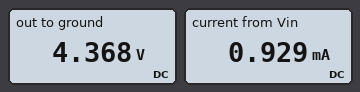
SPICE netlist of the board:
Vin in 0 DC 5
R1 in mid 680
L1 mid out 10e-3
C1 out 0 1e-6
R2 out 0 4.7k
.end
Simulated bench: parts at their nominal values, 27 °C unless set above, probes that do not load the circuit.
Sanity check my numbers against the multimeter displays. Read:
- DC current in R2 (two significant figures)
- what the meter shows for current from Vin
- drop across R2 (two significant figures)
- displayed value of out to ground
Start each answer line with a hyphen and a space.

- 930 µA
- 0.929 mA
- 4.4 V
- 4.368 V
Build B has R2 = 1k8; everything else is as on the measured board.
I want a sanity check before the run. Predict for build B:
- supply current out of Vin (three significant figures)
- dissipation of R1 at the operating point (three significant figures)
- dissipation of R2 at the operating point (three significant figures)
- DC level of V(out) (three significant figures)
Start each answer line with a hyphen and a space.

- 2.02 mA
- 2.76 mW
- 7.32 mW
- 3.63 V
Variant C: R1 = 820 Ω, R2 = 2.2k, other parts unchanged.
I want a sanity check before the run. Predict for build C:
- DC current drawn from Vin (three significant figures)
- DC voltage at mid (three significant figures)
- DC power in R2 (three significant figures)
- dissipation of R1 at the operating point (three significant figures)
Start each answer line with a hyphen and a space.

- 1.66 mA
- 3.64 V
- 6.03 mW
- 2.25 mW
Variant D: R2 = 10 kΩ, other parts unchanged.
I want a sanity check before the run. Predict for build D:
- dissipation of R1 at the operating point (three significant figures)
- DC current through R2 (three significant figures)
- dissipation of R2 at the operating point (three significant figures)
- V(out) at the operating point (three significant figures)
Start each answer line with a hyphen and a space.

- 149 µW
- 468 µA
- 2.19 mW
- 4.68 V
